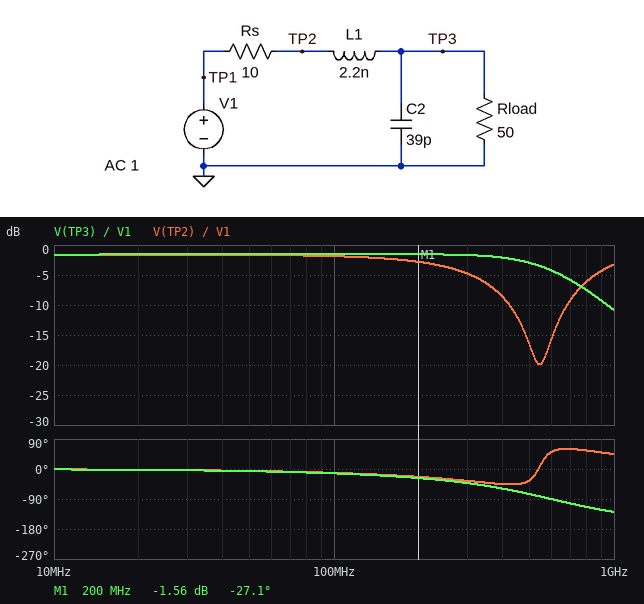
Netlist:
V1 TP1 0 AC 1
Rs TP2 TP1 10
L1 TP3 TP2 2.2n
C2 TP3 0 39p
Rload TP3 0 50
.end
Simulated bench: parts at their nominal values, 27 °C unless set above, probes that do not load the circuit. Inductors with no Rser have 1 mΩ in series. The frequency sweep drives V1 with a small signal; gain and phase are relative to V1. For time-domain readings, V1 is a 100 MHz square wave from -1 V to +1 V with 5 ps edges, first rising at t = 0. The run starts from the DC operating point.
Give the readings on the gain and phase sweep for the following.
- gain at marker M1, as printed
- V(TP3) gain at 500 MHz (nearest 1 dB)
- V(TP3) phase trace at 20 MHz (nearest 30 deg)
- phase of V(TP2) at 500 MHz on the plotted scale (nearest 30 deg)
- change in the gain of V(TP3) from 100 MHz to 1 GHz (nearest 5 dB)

-1.56 dB
-3 dB
0 deg
-30 deg
-10 dB
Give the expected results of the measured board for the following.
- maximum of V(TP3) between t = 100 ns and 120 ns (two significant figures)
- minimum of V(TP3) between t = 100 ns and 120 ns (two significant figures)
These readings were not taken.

930 mV
-930 mV
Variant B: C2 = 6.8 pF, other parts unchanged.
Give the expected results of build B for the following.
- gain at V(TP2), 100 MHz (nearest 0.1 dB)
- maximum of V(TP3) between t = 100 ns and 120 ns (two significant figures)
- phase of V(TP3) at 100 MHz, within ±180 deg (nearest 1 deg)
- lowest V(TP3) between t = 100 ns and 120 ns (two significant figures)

-1.6 dB
1.2 V
-3 deg
-1.2 V
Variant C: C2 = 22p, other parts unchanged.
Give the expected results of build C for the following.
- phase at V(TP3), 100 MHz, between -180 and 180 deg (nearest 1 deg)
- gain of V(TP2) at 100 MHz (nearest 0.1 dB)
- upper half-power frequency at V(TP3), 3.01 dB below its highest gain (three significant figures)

-8 deg
-1.7 dB
909 MHz
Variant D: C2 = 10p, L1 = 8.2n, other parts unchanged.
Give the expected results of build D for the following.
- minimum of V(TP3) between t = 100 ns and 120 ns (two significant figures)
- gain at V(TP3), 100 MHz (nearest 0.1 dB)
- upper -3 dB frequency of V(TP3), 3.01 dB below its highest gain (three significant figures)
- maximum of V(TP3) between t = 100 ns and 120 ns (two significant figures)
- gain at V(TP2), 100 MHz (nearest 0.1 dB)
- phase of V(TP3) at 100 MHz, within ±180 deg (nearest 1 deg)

-1.2 V
-1.4 dB
723 MHz
1.2 V
-1.7 dB
-8 deg
